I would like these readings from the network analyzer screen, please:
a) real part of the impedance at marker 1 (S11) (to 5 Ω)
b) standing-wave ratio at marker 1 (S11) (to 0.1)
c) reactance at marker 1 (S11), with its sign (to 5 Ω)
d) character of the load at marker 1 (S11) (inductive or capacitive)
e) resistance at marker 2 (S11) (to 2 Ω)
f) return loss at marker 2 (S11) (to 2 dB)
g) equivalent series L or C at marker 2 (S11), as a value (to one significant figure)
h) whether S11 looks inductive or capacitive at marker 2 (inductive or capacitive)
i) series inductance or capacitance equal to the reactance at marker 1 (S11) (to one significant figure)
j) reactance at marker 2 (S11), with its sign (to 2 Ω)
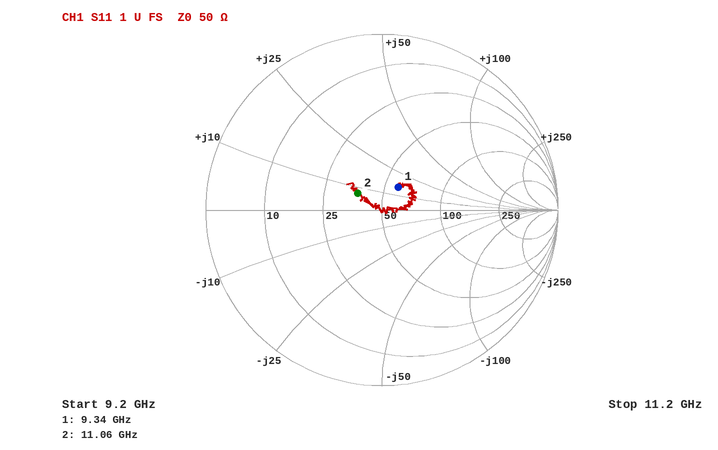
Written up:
60 Ω
1.4
+15 Ω
inductive
38 Ω
16 dB
100 pH
inductive
300 pH
+8 Ω
